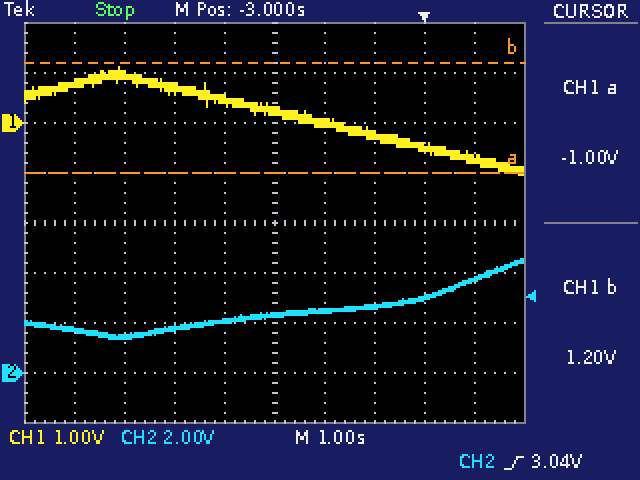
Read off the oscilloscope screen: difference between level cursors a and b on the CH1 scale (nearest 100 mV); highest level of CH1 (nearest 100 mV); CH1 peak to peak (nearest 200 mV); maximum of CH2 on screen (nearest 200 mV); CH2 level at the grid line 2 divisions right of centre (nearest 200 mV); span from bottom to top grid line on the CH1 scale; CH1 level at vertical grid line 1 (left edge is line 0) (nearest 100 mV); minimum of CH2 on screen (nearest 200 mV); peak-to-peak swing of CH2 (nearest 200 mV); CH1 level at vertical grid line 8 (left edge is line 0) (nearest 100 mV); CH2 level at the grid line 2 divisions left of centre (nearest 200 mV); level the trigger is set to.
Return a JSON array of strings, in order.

["2.2 V", "1.1 V", "2.2 V", "4.6 V", "2.6 V", "8 V", "800 mV", "1.4 V", "3.2 V", "-500 mV", "1.8 V", "3.04 V"]
